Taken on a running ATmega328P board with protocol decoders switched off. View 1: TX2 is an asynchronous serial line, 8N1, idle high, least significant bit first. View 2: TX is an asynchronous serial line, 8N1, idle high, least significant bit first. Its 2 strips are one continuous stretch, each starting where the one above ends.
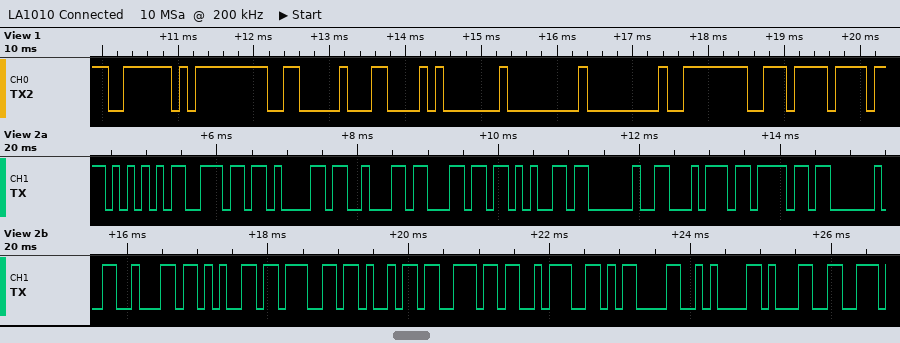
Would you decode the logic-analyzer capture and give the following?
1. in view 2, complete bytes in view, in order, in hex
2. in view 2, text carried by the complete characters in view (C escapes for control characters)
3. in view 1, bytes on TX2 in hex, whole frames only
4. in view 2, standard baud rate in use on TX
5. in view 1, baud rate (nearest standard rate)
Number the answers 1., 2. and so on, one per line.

1. 55 6E 61 62 6C 65 20 74 6F 20 62 65 67 69 6E 3A 0D 0A 31
2. "Unable to begin:\r\n1"
3. 0x7E 0xFF 0x06 0x0C 0x01 0x00 0x00 0xFE 0xEE
4. 9600 baud
5. 9600 baud
